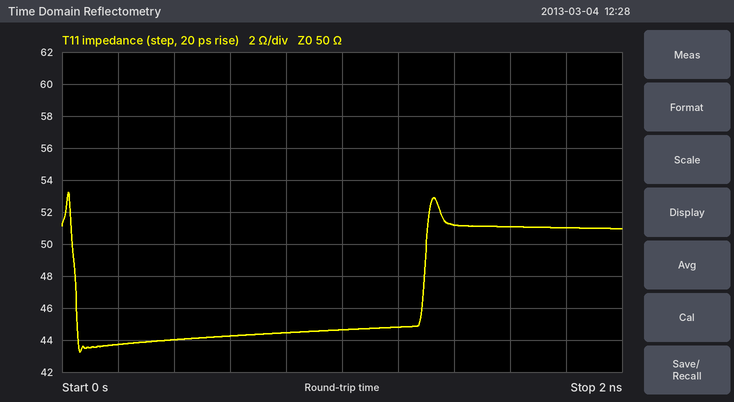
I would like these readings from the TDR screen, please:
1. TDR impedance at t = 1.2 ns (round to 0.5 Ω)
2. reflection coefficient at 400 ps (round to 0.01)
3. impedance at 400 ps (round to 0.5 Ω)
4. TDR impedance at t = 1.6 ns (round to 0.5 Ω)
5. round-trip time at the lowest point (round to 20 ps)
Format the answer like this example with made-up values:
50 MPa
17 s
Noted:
45.0 Ω
-0.06
44.0 Ω
51.0 Ω
60 ps
